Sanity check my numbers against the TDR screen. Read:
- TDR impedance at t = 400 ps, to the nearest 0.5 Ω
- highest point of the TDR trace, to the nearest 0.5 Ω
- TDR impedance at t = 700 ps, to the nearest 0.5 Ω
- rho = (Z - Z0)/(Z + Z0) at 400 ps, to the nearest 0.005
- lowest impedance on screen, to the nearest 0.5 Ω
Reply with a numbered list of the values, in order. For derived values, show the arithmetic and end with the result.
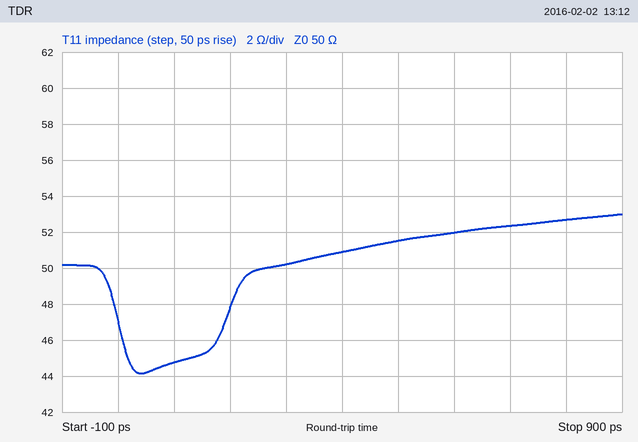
1. 51.0 Ω
2. 53.0 Ω
3. 52.5 Ω
4. (51 − 50)/(51 + 50) ≈ +0.010
5. 44.0 Ω
